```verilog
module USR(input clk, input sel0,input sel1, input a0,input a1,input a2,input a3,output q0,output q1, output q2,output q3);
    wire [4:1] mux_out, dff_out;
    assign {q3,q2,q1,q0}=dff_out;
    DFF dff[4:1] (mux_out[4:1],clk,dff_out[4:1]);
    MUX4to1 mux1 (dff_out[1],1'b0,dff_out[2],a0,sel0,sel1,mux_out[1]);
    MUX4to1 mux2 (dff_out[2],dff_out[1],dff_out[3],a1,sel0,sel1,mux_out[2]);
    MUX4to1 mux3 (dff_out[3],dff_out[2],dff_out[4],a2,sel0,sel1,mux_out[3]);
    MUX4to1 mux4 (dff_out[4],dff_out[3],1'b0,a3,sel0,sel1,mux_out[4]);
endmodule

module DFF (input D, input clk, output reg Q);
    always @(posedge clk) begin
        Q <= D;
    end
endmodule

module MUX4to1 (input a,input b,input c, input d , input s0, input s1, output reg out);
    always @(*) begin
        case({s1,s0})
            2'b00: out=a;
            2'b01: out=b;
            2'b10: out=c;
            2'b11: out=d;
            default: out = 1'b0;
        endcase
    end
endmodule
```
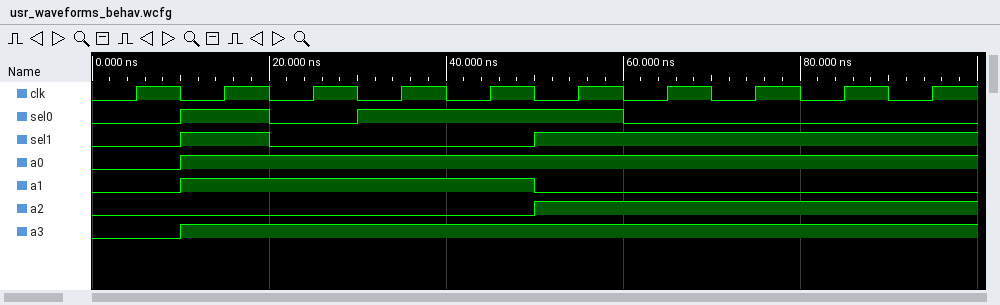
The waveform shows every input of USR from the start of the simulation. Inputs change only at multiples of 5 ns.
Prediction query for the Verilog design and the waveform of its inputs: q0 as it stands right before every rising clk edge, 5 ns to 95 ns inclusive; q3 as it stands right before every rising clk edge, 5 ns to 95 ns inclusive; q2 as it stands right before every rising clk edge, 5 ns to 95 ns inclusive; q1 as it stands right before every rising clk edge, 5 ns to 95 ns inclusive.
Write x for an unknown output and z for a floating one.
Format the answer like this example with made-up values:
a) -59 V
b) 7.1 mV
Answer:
a) x x 1 1 0 0 1 0 1 1
b) x x 1 1 0 1 1 0 0 0
c) x x 0 0 1 1 1 1 0 0
d) x x 1 1 1 0 0 1 1 0
